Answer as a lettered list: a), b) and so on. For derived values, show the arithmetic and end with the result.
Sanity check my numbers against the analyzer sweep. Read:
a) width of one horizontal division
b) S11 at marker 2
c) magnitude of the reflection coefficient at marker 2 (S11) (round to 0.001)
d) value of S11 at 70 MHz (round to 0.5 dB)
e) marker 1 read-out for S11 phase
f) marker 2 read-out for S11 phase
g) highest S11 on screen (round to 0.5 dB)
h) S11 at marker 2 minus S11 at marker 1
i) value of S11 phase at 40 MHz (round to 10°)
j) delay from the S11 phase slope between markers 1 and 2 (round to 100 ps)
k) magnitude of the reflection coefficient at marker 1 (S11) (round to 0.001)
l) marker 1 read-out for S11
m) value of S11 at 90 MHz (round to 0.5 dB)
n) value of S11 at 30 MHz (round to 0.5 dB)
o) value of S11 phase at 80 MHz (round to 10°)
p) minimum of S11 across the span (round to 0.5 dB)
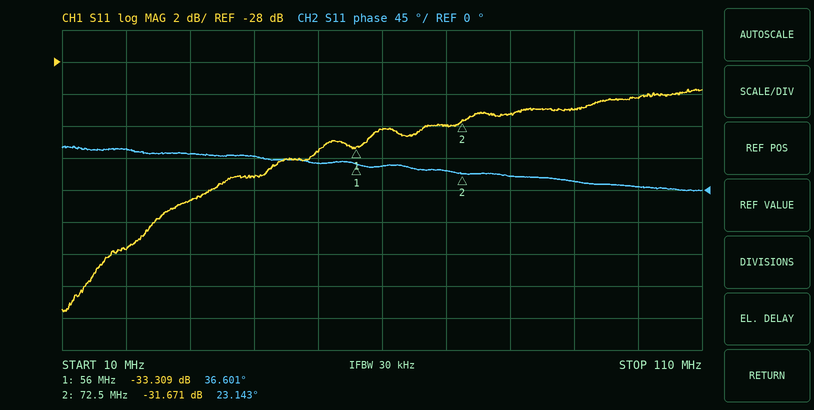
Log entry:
a) 10 MHz
b) -31.671 dB
c) 10^(-31.671/20) ≈ 0.026
d) -32.0 dB
e) 36.601°
f) 23.143°
g) -29.5 dB
h) -31.671 − (-33.309) = 1.638 dB
i) 50°
j) −(23.143° − (36.601°))/(360° × 16.5 MHz) ≈ 2.3 ns
k) 10^(-33.309/20) ≈ 0.022
l) -33.309 dB
m) -31.0 dB
n) -36.5 dB
o) 20°
p) -43.5 dB
